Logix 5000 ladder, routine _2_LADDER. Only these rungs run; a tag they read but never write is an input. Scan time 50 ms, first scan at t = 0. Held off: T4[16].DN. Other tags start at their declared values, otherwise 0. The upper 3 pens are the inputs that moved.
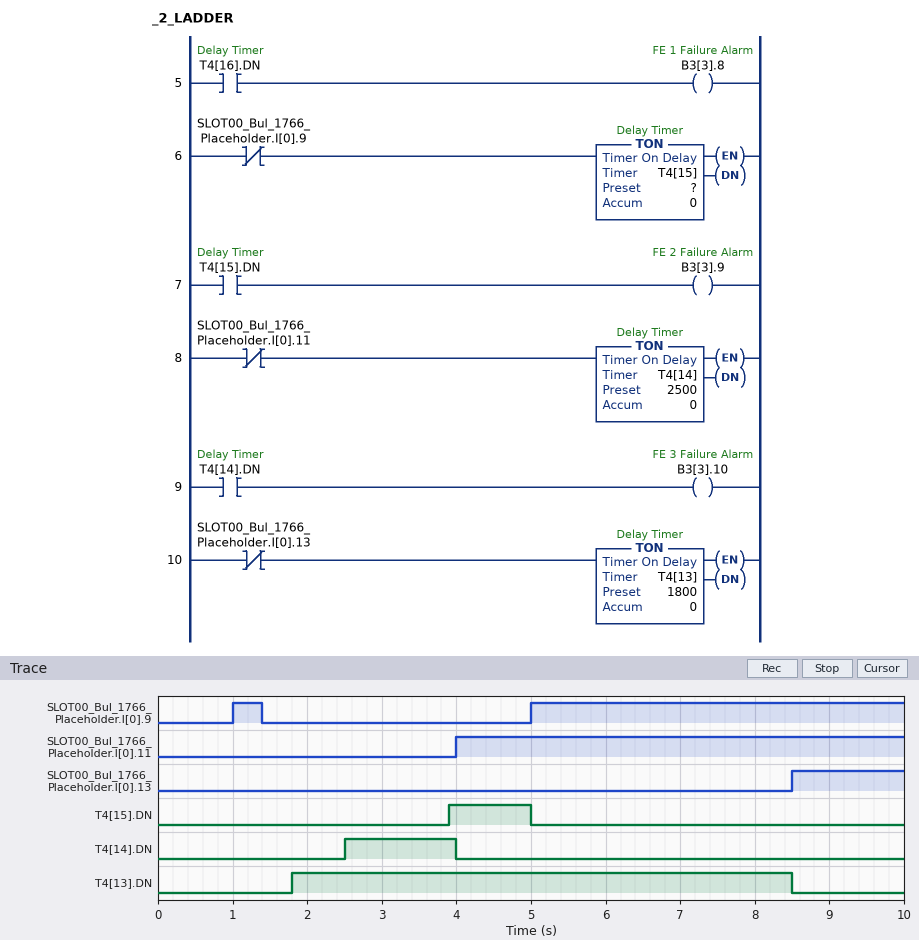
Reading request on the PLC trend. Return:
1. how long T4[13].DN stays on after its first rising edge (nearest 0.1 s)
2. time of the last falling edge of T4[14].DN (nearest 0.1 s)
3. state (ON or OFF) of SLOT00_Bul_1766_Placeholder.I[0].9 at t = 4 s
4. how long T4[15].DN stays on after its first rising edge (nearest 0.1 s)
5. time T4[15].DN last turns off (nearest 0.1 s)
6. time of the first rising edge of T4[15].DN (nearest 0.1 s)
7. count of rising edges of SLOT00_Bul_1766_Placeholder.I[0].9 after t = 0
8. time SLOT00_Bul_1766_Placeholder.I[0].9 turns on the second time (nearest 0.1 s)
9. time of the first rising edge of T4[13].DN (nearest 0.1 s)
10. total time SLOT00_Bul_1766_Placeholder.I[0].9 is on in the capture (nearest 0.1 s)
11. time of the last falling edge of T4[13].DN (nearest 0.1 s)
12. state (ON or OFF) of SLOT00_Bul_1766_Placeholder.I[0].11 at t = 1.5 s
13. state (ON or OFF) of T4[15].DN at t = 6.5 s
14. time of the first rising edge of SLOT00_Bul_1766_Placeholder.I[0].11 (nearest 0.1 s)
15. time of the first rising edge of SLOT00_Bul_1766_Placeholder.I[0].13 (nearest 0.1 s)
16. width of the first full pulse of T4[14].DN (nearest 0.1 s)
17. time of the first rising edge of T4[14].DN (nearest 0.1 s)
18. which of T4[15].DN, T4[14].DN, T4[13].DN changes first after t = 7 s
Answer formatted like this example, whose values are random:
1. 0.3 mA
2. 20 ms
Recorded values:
1. 6.7 s
2. 4.0 s
3. OFF
4. 1.1 s
5. 5.0 s
6. 3.9 s
7. 2
8. 5.0 s
9. 1.8 s
10. 5.4 s
11. 8.5 s
12. OFF
13. OFF
14. 4.0 s
15. 8.5 s
16. 1.5 s
17. 2.5 s
18. T4[13].DN
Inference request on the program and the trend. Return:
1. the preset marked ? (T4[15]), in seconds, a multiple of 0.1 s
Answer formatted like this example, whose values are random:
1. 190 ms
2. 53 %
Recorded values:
1. 2.5 s
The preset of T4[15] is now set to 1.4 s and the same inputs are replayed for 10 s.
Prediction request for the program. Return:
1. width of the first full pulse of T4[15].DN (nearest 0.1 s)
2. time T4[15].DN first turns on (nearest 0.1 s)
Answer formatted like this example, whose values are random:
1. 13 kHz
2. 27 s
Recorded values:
1. 2.2 s
2. 2.8 s
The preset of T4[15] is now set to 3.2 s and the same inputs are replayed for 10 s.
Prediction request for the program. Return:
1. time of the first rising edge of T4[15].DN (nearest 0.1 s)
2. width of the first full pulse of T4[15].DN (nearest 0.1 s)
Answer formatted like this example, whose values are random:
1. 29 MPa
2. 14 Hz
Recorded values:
1. 4.6 s
2. 0.4 s
